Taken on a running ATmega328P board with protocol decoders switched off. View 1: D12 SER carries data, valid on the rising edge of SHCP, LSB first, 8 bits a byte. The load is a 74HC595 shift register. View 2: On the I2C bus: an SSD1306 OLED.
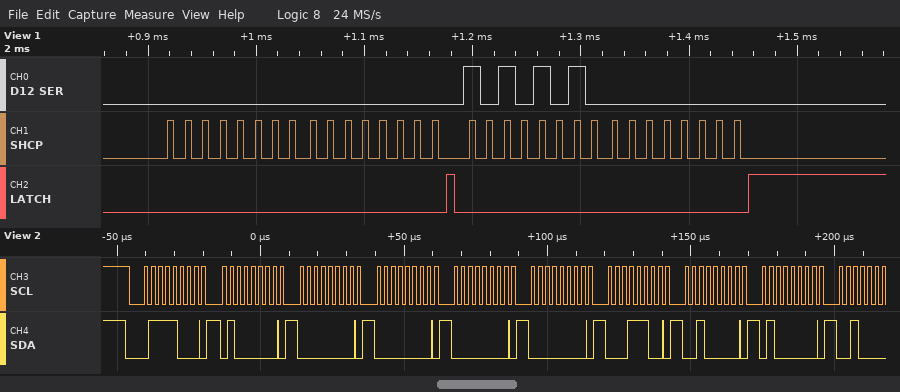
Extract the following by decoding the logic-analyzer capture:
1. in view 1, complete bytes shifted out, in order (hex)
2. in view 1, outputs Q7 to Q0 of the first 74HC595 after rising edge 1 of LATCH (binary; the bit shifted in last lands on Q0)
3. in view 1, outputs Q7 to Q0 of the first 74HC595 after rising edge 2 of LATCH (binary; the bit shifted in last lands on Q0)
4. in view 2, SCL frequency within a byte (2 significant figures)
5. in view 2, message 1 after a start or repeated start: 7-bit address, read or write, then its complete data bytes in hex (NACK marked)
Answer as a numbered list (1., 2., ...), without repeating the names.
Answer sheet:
1. 00 00 55 00
2. 00000000
3. 00000000
4. 400 kHz
5. 0x3C write: 40 00 00 00 00 1C 20 40
